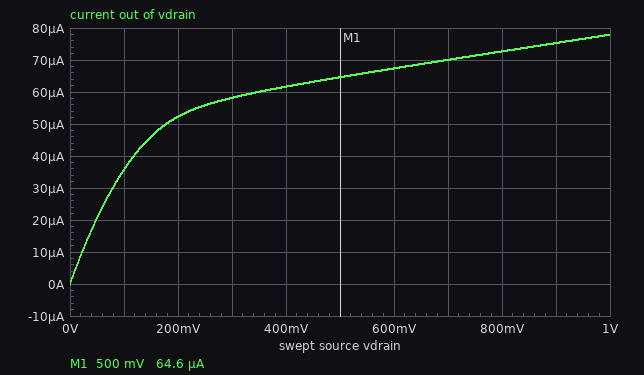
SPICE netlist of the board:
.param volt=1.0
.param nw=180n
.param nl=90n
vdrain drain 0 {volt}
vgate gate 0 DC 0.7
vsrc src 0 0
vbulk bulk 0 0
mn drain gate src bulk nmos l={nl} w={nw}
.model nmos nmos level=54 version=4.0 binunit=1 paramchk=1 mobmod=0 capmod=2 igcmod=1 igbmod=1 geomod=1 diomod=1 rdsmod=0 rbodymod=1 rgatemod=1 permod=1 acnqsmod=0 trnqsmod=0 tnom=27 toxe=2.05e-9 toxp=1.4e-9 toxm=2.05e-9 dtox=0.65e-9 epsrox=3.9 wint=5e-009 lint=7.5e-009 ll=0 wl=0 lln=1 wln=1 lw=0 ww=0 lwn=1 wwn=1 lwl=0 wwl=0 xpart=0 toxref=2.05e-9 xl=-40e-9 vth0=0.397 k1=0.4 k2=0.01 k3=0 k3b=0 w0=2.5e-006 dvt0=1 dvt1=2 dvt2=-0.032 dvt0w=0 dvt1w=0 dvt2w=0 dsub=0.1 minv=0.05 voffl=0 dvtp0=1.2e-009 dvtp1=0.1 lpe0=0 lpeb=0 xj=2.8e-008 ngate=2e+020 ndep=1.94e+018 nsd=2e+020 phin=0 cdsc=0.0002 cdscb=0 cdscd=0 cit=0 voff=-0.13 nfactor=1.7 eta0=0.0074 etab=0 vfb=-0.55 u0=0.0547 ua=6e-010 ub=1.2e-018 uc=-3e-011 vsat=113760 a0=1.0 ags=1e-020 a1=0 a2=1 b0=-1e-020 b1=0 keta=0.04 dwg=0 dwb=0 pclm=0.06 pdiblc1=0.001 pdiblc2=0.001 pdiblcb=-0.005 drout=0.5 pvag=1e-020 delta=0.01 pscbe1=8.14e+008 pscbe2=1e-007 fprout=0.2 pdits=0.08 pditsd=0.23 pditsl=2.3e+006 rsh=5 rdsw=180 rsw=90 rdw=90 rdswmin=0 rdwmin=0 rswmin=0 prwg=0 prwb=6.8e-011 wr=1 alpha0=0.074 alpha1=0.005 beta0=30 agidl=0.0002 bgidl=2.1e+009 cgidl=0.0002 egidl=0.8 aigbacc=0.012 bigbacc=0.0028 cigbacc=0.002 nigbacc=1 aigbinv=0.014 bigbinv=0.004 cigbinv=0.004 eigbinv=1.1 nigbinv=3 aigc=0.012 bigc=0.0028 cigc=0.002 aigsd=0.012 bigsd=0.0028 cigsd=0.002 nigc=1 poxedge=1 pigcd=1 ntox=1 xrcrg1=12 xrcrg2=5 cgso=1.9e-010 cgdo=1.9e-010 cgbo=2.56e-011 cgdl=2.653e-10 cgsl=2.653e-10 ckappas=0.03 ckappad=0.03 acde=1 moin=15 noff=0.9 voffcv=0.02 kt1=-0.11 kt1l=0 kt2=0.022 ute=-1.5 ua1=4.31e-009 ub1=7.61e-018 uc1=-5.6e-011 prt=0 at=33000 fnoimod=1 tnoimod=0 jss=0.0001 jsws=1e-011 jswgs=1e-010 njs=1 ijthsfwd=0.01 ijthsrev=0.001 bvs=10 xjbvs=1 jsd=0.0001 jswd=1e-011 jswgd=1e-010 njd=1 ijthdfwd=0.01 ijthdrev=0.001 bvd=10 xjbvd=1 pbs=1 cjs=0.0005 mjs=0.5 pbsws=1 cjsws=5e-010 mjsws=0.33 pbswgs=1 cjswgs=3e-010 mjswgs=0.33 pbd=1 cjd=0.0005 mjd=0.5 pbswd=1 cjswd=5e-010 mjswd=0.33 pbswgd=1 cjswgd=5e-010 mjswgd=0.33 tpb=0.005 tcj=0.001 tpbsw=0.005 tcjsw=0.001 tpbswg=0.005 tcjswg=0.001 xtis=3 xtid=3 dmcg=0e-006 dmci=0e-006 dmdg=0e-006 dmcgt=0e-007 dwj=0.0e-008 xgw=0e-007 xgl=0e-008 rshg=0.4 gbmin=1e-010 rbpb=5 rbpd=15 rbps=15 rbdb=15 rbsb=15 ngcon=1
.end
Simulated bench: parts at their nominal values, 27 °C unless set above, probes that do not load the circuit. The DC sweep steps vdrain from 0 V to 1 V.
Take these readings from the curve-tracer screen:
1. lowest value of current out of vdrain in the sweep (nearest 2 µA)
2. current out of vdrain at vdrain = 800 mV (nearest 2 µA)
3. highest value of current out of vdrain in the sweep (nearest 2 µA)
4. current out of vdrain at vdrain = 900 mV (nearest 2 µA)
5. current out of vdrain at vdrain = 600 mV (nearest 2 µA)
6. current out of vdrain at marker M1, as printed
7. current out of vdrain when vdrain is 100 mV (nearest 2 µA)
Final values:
0 A
72 µA
78 µA
76 µA
68 µA
64.6 µA
36 µA
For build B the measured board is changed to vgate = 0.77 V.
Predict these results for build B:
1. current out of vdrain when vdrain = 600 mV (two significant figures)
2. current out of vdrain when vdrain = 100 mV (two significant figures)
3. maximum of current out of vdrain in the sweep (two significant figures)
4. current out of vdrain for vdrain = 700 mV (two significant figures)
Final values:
82 µA
41 µA
93 µA
85 µA
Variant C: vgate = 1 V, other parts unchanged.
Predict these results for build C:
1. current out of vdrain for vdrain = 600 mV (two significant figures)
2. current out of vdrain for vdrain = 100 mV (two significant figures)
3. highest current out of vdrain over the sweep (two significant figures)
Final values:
130 µA
52 µA
140 µA
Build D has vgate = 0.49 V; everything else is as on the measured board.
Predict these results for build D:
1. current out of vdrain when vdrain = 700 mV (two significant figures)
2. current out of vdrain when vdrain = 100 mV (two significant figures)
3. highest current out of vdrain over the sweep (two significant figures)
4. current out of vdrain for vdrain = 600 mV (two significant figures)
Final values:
26 µA
13 µA
32 µA
24 µA
